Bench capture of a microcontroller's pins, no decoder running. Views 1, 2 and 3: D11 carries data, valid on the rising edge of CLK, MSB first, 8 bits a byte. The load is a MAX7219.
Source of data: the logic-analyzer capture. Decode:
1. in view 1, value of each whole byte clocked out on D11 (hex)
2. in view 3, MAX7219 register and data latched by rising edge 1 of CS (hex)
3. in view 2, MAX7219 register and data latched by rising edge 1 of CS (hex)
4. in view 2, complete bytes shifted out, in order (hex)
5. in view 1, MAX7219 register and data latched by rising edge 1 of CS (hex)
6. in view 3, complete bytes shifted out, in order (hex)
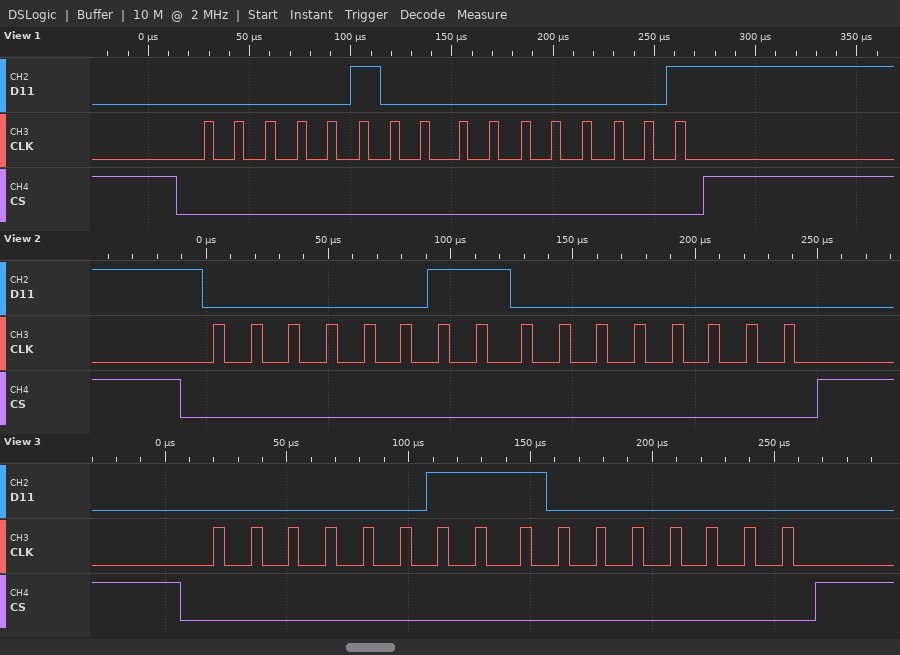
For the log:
04 01
register 0x3, data 0x80
register 0x3, data 0x00
03 00
register 0x4, data 0x01
03 80
